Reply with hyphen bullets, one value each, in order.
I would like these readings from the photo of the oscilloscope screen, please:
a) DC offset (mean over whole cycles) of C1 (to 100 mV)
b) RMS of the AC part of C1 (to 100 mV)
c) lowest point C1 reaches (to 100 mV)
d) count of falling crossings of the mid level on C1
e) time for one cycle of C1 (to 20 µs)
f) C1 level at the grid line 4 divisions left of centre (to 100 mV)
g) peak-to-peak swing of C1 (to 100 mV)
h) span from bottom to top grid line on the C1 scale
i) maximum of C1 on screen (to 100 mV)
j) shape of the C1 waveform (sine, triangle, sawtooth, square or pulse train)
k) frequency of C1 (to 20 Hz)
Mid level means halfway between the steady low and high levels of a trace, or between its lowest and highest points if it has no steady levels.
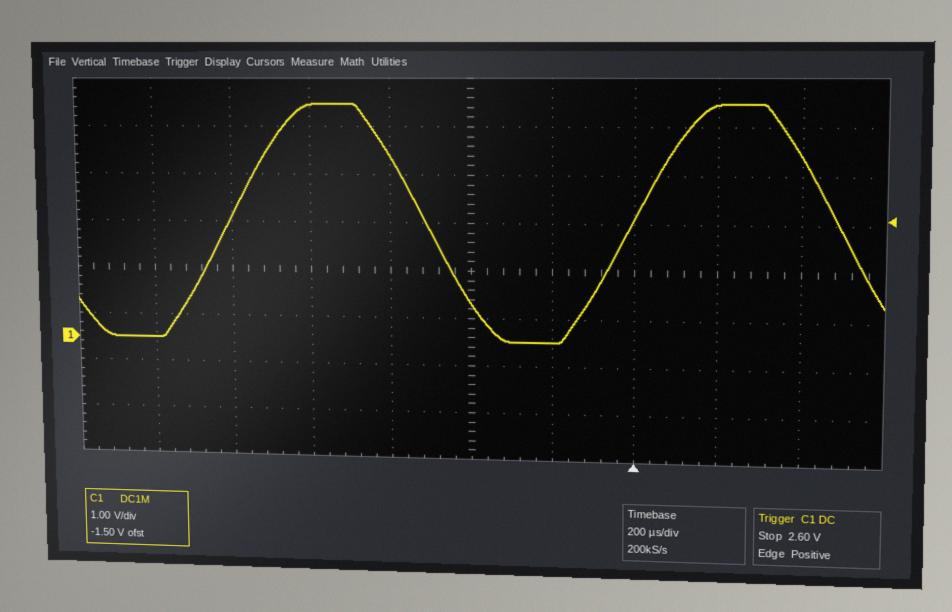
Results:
- 2.5 V
- 1.8 V
- 0.0 V
- 2
- 1.00 ms
- 0.0 V
- 5.0 V
- 8 V
- 5.0 V
- sine
- 1.00 kHz
